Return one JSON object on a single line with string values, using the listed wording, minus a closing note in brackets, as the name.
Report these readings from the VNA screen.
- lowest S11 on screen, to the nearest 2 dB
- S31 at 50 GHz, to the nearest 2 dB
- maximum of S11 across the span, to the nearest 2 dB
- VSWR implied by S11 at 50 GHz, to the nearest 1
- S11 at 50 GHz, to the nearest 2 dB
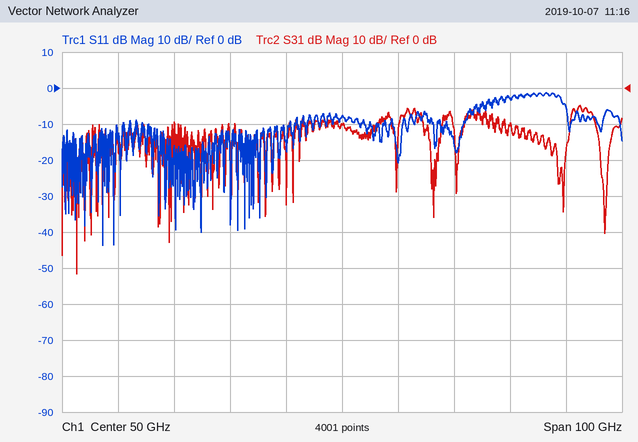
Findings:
{"lowest S11 on screen, to the nearest 2 dB": "-44 dB", "S31 at 50 GHz, to the nearest 2 dB": "-10 dB", "maximum of S11 across the span, to the nearest 2 dB": "-2 dB", "VSWR implied by S11 at 50 GHz, to the nearest 1": "2", "S11 at 50 GHz, to the nearest 2 dB": "-8 dB"}
